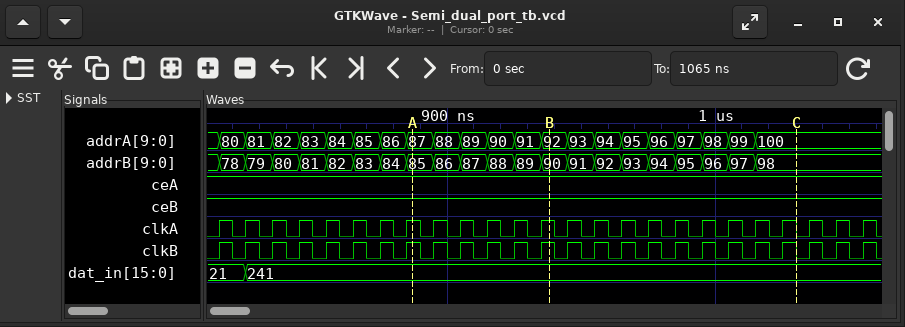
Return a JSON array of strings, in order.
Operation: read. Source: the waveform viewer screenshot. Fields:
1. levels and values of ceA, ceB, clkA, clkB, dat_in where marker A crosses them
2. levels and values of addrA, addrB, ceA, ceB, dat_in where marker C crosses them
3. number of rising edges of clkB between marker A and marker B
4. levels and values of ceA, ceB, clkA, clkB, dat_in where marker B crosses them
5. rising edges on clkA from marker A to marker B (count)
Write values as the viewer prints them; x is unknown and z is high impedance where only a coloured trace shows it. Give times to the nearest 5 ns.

["ceA=1, ceB=1, clkA=1, clkB=1, dat_in=241", "addrA=100, addrB=98, ceA=1, ceB=1, dat_in=241", "5", "ceA=1, ceB=1, clkA=1, clkB=1, dat_in=241", "5"]
